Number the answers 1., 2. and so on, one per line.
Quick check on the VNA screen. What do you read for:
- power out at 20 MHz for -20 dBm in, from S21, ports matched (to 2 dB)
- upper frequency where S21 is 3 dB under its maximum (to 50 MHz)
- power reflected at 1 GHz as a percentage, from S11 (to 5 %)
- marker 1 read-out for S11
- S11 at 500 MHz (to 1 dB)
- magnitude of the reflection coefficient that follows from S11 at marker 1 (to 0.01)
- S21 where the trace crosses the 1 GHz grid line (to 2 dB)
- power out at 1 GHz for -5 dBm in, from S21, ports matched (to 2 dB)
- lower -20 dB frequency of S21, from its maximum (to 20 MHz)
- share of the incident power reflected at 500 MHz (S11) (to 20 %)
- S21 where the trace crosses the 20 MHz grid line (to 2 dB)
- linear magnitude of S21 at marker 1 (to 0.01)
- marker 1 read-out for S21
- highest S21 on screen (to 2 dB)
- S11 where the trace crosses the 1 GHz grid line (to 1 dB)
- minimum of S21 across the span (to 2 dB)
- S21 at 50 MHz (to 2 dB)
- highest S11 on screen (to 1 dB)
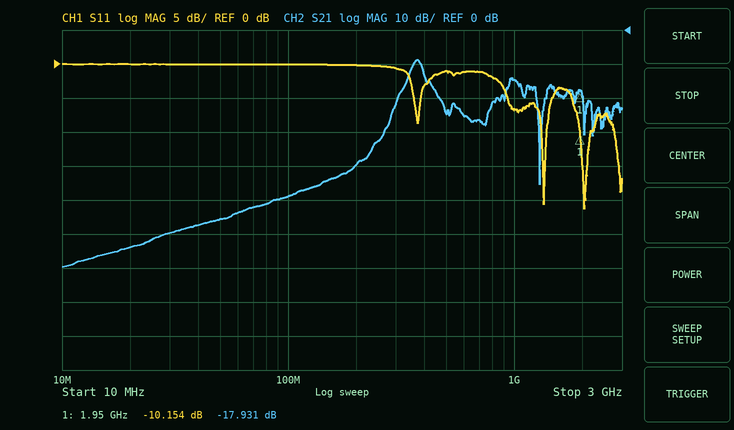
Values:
1. -84 dBm
2. 400 MHz
3. 20 %
4. -10.154 dB
5. -1 dB
6. 0.31
7. -14 dB
8. -20 dBm
9. 280 MHz
10. 80 %
11. -64 dB
12. 0.13
13. -17.931 dB
14. -8 dB
15. -7 dB
16. -70 dB
17. -56 dB
18. 0 dB
